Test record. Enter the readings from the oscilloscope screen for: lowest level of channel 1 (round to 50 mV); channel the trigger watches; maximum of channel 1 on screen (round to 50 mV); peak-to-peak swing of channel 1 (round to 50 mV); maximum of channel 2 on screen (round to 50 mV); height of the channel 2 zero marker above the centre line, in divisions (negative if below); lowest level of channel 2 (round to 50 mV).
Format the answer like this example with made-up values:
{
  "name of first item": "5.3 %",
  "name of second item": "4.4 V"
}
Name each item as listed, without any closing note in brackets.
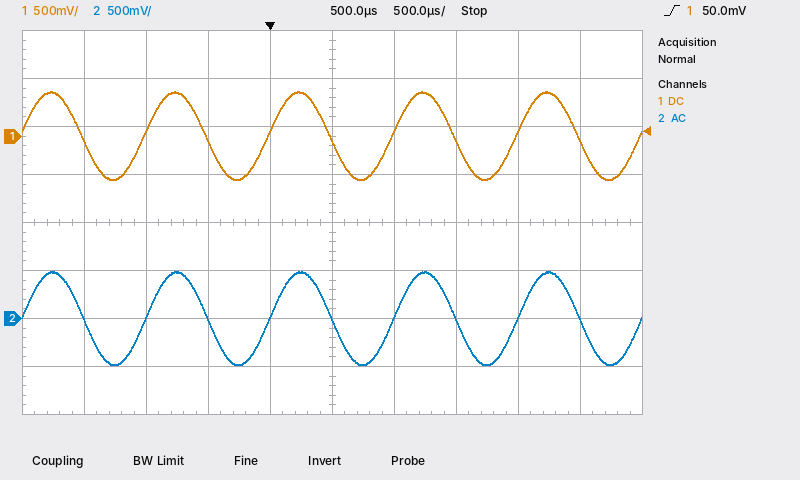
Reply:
{
  "lowest level of channel 1": "-450 mV",
  "channel the trigger watches": "channel 1",
  "maximum of channel 1 on screen": "450 mV",
  "peak-to-peak swing of channel 1": "900 mV",
  "maximum of channel 2 on screen": "500 mV",
  "height of the channel 2 zero marker above the centre line, in divisions": "-2.0 div",
  "lowest level of channel 2": "-500 mV"
}
